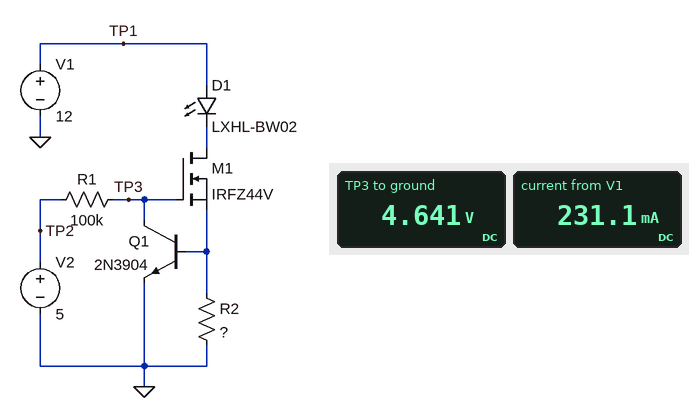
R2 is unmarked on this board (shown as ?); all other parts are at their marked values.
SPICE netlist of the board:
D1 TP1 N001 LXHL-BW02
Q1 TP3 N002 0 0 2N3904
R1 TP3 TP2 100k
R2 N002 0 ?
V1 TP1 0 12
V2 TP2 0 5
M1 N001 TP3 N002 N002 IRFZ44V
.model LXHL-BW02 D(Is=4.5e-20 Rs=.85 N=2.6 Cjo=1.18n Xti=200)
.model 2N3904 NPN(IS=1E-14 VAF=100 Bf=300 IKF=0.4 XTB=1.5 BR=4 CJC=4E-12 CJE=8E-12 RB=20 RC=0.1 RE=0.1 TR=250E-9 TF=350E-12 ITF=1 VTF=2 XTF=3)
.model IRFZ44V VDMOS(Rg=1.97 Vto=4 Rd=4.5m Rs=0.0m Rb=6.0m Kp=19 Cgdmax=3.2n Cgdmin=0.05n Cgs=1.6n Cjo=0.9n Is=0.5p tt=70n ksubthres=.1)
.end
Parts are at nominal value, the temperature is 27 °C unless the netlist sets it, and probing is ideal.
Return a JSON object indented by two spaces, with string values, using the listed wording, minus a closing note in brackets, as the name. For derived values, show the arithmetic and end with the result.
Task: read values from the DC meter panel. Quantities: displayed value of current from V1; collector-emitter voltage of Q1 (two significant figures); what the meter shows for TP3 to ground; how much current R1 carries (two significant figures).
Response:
{
  "displayed value of current from V1": "231.1 mA",
  "collector-emitter voltage of Q1": "4.641 V = 4.6 V",
  "what the meter shows for TP3 to ground": "4.641 V",
  "how much current R1 carries": "(5 V - 4.641 V) / 100 kΩ = 3.6 µA"
}
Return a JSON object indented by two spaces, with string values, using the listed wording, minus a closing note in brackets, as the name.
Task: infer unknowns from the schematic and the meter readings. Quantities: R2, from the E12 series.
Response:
{
  "R2, from the E12 series": "2.2 Ω"
}
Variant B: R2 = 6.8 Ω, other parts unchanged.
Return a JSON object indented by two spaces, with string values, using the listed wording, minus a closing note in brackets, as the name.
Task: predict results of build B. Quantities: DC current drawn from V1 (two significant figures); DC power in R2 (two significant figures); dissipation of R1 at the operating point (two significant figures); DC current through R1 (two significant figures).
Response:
{
  "DC current drawn from V1": "76 mA",
  "DC power in R2": "39 mW",
  "dissipation of R1 at the operating point": "2.0 µW",
  "DC current through R1": "4.5 µA"
}
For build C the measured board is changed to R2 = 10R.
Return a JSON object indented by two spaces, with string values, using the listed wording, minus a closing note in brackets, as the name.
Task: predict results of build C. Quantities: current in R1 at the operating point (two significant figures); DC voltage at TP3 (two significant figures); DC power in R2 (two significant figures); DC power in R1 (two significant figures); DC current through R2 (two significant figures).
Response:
{
  "current in R1 at the operating point": "4.8 µA",
  "DC voltage at TP3": "4.5 V",
  "DC power in R2": "27 mW",
  "DC power in R1": "2.3 µW",
  "DC current through R2": "52 mA"
}
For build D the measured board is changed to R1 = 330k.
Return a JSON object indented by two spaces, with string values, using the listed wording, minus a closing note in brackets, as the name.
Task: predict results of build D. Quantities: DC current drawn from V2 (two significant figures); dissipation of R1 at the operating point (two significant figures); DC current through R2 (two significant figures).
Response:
{
  "DC current drawn from V2": "1.2 µA",
  "dissipation of R1 at the operating point": "470 nW",
  "DC current through R2": "220 mA"
}
